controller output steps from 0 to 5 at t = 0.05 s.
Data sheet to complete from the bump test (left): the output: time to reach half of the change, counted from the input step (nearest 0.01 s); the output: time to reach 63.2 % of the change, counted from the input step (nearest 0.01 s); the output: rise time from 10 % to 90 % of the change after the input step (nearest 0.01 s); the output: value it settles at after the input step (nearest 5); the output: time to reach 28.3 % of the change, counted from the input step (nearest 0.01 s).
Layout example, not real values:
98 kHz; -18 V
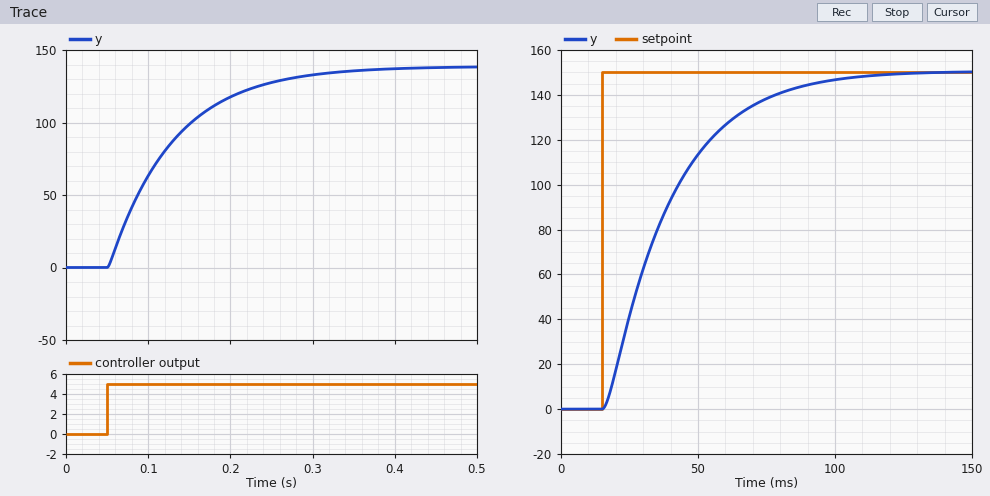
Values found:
0.06 s; 0.08 s; 0.17 s; 140; 0.03 s
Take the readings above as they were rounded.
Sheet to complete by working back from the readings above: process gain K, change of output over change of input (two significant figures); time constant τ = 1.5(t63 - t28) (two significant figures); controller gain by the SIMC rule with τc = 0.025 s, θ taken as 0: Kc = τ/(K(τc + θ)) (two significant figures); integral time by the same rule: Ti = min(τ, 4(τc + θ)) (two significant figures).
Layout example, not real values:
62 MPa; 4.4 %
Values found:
28; 0.075 s; 0.11; 0.075 s
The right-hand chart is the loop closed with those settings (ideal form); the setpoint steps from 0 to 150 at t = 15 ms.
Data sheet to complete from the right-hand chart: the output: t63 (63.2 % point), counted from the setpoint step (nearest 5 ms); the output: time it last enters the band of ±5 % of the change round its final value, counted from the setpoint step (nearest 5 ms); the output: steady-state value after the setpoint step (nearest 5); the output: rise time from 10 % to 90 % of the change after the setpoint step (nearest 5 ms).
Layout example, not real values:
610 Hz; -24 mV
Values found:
25 ms; 70 ms; 150; 50 ms
